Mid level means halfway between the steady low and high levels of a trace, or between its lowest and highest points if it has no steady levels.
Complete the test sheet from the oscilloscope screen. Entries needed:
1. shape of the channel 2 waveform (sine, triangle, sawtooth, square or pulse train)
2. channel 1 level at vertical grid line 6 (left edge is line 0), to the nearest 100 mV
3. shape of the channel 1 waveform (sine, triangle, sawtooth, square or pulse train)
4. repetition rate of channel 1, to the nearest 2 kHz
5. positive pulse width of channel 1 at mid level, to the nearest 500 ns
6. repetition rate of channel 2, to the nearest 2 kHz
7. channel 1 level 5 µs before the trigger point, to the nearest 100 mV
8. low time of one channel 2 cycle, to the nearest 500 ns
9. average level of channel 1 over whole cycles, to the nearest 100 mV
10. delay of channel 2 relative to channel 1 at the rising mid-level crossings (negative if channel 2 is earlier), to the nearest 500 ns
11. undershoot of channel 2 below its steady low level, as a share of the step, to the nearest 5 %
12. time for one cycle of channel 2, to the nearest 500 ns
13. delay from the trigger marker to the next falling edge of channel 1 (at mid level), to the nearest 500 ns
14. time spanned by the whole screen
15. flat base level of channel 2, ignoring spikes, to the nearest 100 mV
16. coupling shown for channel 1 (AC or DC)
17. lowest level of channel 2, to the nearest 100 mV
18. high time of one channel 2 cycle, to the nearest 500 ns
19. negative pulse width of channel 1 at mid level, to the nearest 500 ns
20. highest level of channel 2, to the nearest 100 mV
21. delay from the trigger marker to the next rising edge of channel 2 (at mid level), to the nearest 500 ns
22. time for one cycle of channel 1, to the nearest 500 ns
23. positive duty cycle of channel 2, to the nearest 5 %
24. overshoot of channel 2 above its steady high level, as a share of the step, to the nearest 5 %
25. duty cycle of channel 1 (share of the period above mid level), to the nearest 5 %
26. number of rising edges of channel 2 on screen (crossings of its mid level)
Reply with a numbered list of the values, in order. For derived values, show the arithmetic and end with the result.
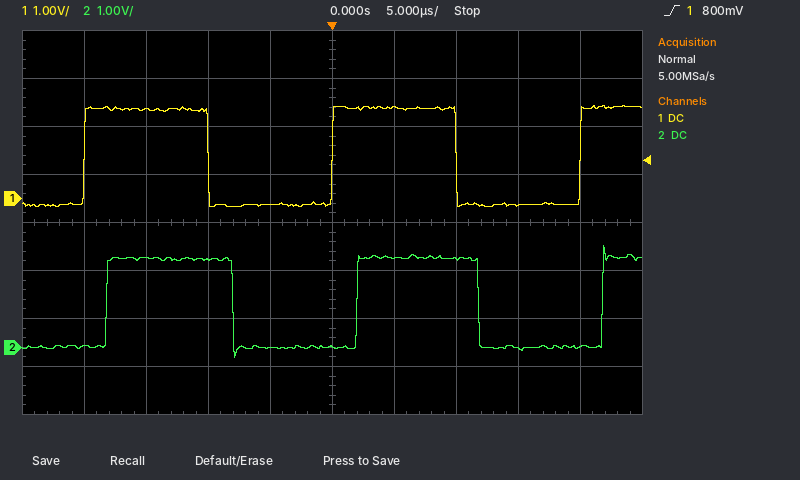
1. square
2. 1.9 V
3. square
4. 1 / 20.0 µs ≈ 50 kHz
5. 10.0 µs
6. 1 / 20.0 µs ≈ 50 kHz
7. -100 mV
8. 10.0 µs
9. -100 mV + 0.5 × (1.9 V − (-100 mV)) ≈ 900 mV
10. +2.0 µs
11. 10 %
12. 20.0 µs
13. 10.0 µs
14. 50 µs
15. 0.0 V
16. DC
17. -200 mV
18. 10.0 µs
19. 10.0 µs
20. 2.1 V
21. 2.0 µs
22. 20.0 µs
23. 10.0 µs / 20.0 µs ≈ 50 %
24. 15 %
25. 10.0 µs / 20.0 µs ≈ 50 %
26. 3
